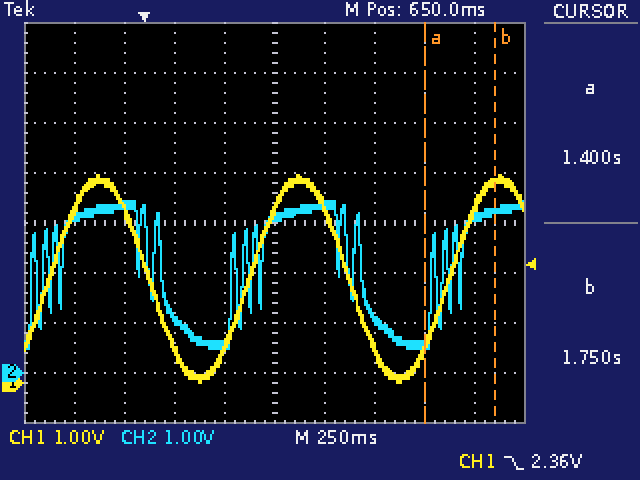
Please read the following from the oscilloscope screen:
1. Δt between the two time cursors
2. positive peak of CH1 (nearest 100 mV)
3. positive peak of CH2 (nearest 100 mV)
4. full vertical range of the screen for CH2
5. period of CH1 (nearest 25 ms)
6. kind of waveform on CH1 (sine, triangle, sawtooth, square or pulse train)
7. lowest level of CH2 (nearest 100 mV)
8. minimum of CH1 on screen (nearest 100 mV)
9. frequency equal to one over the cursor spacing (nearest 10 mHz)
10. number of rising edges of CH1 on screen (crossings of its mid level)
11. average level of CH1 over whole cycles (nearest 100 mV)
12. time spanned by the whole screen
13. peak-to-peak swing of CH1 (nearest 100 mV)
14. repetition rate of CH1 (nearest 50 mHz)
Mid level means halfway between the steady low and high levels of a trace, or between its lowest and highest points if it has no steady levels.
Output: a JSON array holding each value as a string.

["350 ms", "4.2 V", "3.4 V", "8 V", "1.000 s", "sine", "500 mV", "0.0 V", "2.86 Hz", "3", "2.1 V", "2.5 s", "4.2 V", "1.00 Hz"]
